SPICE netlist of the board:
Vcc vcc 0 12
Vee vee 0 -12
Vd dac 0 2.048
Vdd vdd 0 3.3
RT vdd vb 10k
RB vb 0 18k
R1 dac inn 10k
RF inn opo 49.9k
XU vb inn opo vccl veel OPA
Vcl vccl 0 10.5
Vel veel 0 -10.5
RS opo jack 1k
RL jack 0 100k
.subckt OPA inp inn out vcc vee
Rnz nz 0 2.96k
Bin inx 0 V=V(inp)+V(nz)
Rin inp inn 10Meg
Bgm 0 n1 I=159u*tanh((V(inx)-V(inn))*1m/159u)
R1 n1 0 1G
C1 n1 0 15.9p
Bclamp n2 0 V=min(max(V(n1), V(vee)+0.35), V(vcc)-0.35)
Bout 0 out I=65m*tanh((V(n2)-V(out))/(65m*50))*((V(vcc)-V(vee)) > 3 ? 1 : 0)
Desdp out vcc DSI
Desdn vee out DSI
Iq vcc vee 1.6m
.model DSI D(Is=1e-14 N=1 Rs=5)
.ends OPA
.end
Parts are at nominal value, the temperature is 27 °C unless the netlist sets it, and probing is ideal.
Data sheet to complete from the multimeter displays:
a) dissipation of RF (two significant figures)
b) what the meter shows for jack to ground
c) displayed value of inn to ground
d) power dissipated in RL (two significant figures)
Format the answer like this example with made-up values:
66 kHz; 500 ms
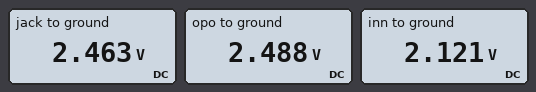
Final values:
2.7 µW; 2.463 V; 2.121 V; 61 µW
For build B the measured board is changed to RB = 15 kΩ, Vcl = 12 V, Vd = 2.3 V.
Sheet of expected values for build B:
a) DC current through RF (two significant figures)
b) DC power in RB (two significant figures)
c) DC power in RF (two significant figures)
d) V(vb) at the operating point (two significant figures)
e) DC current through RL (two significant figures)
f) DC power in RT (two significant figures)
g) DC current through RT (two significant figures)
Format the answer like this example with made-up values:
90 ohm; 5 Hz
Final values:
32 µA; 260 µW; 51 µW; 2.0 V; 3.8 µA; 170 µW; 130 µA
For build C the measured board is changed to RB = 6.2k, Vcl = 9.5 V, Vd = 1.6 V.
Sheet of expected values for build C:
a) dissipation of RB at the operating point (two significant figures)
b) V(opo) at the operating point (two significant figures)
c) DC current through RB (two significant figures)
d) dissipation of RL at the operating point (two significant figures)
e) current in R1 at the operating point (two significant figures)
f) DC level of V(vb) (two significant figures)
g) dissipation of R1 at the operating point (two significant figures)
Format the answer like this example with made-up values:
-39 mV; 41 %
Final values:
260 µW; -420 mV; 200 µA; 1.7 µW; 34 µA; 1.3 V; 11 µW
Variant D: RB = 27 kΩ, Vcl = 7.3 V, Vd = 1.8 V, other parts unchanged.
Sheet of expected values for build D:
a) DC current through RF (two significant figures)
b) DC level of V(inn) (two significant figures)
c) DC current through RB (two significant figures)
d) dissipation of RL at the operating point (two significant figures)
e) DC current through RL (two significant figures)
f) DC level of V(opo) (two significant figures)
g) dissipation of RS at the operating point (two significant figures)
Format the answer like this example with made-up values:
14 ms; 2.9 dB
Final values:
61 µA; 2.4 V; 89 µA; 290 µW; 54 µA; 5.4 V; 2.9 µW
